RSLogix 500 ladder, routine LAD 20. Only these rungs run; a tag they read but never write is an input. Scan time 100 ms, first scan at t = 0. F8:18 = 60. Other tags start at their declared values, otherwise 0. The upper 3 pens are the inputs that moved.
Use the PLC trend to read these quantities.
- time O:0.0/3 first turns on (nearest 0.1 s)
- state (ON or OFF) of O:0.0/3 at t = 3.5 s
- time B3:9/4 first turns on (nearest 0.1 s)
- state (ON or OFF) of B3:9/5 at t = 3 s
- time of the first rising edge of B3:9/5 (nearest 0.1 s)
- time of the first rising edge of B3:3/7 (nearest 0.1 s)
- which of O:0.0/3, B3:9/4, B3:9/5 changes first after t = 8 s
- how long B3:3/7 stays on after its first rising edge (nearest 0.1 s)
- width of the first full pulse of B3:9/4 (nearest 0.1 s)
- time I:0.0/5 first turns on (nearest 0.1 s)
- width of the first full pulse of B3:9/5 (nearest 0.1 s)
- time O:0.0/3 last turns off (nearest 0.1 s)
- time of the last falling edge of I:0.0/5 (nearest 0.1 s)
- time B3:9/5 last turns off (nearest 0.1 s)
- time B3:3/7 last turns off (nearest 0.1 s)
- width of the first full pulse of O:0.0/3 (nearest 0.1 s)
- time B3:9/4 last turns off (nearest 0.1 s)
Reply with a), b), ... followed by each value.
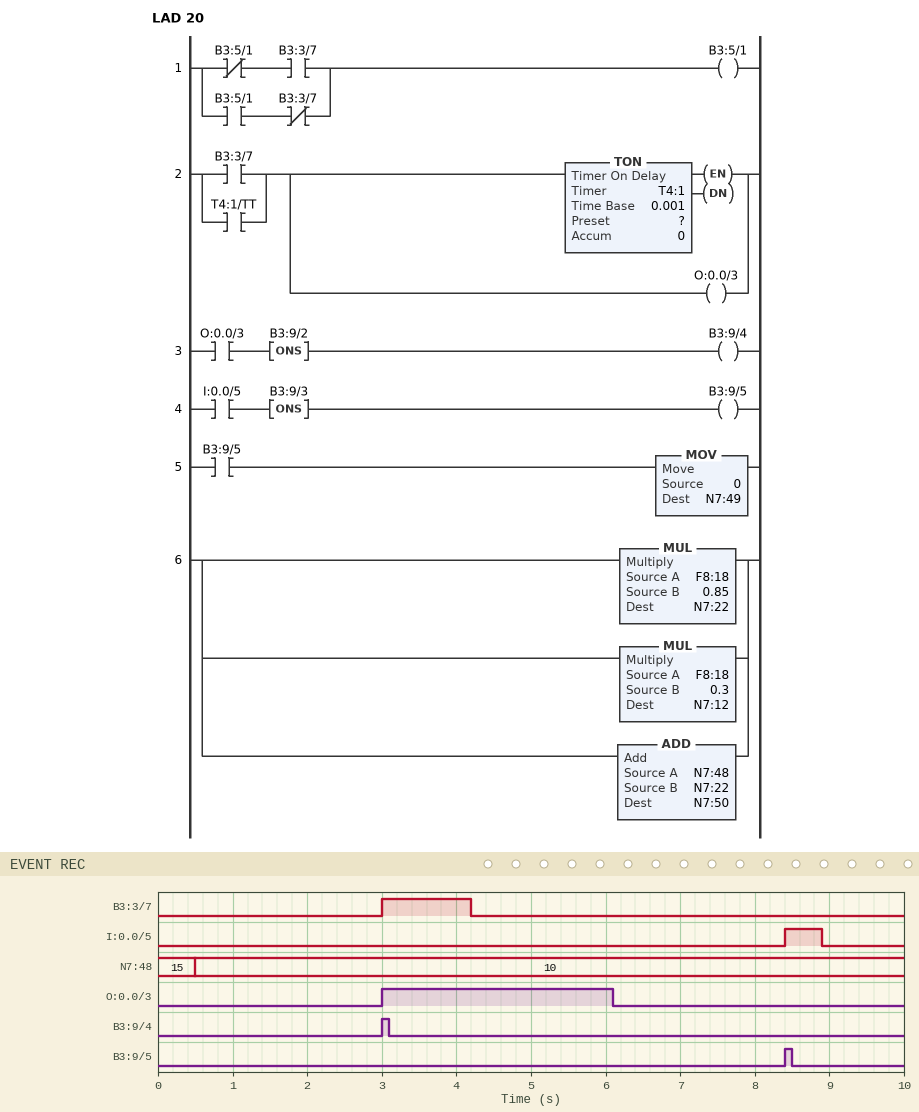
a) 3.0 s
b) ON
c) 3.0 s
d) OFF
e) 8.4 s
f) 3.0 s
g) B3:9/5
h) 1.2 s
i) 0.1 s
j) 8.4 s
k) 0.1 s
l) 6.1 s
m) 8.9 s
n) 8.5 s
o) 4.2 s
p) 3.1 s
q) 3.1 s
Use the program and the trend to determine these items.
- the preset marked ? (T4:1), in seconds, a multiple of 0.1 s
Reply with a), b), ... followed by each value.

a) 3.0 s
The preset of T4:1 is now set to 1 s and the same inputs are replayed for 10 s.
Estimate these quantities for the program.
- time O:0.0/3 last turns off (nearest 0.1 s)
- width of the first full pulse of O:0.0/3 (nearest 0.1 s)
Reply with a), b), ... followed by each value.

a) 4.2 s
b) 1.2 s
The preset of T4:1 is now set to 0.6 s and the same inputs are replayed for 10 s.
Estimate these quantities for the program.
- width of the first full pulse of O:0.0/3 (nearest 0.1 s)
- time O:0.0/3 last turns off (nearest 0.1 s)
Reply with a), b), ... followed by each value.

a) 1.2 s
b) 4.2 s
